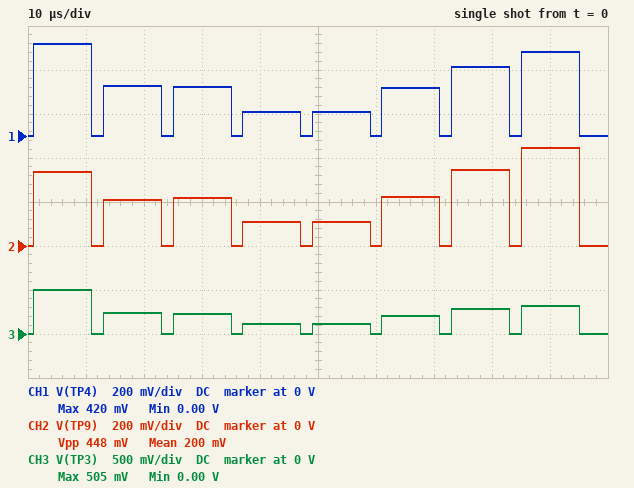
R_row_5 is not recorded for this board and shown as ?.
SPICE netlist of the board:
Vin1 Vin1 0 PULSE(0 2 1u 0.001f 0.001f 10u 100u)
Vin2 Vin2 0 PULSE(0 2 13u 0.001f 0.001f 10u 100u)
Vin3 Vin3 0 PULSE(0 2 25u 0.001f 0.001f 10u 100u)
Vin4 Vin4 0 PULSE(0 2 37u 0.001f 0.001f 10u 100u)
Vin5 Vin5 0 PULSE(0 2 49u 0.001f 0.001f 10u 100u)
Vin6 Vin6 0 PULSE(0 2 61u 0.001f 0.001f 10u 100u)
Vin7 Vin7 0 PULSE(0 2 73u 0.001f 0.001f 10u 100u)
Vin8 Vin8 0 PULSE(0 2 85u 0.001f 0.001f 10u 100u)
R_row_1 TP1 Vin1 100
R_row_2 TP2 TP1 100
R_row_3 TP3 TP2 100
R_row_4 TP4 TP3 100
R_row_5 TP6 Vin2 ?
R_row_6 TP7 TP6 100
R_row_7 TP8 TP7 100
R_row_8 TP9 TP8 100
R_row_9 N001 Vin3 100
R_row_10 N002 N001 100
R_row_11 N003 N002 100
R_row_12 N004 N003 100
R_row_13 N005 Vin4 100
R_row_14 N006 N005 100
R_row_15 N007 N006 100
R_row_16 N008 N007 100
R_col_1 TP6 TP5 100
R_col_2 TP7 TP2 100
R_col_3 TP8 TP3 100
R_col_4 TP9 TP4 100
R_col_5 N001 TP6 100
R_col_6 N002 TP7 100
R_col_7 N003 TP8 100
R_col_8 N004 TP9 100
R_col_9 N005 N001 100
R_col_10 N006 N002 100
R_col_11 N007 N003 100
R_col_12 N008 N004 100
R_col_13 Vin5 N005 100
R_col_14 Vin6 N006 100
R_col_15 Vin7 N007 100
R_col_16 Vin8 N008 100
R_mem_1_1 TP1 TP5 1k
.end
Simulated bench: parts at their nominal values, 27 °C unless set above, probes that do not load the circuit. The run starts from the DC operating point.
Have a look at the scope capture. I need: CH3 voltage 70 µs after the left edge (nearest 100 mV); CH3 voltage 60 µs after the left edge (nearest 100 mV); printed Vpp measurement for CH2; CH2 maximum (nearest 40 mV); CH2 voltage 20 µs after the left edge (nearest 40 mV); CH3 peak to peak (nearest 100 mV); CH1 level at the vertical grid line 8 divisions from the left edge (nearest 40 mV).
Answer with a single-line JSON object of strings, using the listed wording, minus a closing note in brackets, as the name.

{"CH3 voltage 70 µs after the left edge": "200 mV", "CH3 voltage 60 µs after the left edge": "0 V", "printed Vpp measurement for CH2": "448 mV", "CH2 maximum": "440 mV", "CH2 voltage 20 µs after the left edge": "200 mV", "CH3 peak to peak": "500 mV", "CH1 level at the vertical grid line 8 divisions from the left edge": "320 mV"}
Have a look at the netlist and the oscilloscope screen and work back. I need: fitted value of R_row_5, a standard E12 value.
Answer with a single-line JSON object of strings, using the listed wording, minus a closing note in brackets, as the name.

{"fitted value of R_row_5, a standard E12 value": "150 Ω"}
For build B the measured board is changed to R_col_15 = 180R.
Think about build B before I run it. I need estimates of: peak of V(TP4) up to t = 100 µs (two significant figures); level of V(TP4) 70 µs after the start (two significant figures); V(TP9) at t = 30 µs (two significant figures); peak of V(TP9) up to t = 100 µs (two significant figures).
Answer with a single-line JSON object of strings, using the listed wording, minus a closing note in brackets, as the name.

{"peak of V(TP4) up to t = 100 µs": "430 mV", "level of V(TP4) 70 µs after the start": "240 mV", "V(TP9) at t = 30 µs": "230 mV", "peak of V(TP9) up to t = 100 µs": "480 mV"}
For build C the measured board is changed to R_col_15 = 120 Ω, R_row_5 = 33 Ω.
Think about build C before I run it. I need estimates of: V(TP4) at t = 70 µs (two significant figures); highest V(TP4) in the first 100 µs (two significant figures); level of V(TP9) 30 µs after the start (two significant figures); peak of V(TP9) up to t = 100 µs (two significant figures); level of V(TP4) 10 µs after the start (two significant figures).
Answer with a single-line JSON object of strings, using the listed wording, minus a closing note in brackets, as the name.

{"V(TP4) at t = 70 µs": "200 mV", "highest V(TP4) in the first 100 µs": "460 mV", "level of V(TP9) 30 µs after the start": "160 mV", "peak of V(TP9) up to t = 100 µs": "440 mV", "level of V(TP4) 10 µs after the start": "380 mV"}
